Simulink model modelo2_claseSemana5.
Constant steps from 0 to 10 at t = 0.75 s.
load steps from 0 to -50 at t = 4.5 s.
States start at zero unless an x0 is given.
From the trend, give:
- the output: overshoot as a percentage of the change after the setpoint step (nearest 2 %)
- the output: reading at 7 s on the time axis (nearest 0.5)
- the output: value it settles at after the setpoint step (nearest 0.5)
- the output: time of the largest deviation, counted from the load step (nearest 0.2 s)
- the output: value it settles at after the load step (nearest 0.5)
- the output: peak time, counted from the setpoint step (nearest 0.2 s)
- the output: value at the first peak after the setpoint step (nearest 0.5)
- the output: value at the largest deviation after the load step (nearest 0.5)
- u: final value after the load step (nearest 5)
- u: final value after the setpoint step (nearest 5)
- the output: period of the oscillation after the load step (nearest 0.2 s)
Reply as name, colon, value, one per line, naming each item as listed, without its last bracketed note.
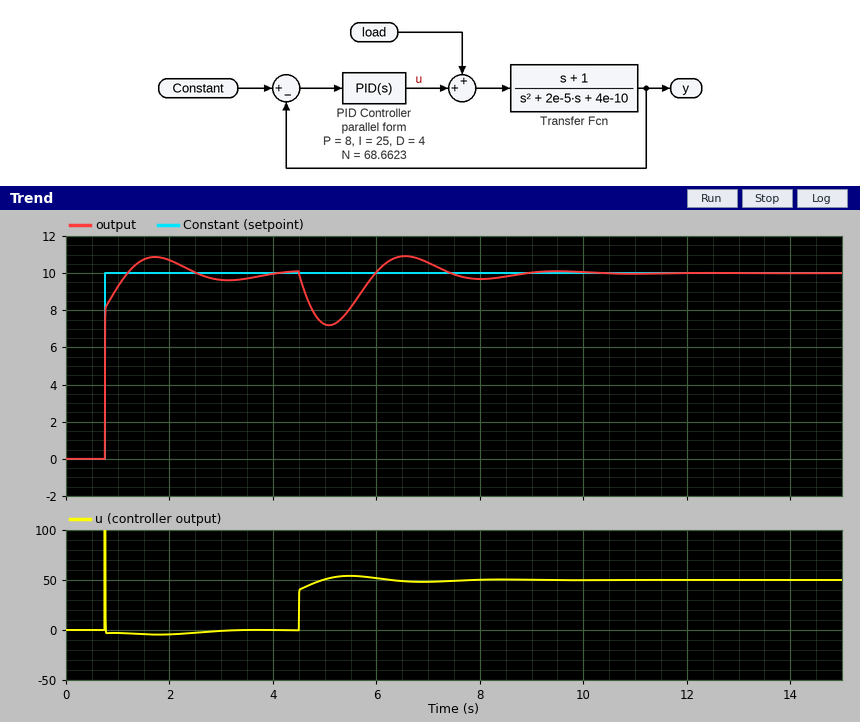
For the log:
the output: overshoot as a percentage of the change after the setpoint step: 8 %
the output: reading at 7 s on the time axis: 10.5
the output: value it settles at after the setpoint step: 10.0
the output: time of the largest deviation, counted from the load step: 0.6 s
the output: value it settles at after the load step: 10.0
the output: peak time, counted from the setpoint step: 1.0 s
the output: value at the first peak after the setpoint step: 11.0
the output: value at the largest deviation after the load step: 7.0
u: final value after the load step: 50
u: final value after the setpoint step: 0
the output: period of the oscillation after the load step: 3.0 s
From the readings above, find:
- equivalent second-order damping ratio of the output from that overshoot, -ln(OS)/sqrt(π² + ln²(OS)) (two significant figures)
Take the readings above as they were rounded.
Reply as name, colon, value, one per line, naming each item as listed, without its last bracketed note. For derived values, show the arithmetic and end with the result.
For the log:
equivalent second-order damping ratio of the output from that overshoot, -ln(OS)/sqrt(π² + ln²(OS)): ln(0.08) = -2.526; 2.526 / sqrt(9.870 + 6.379) = 0.63
